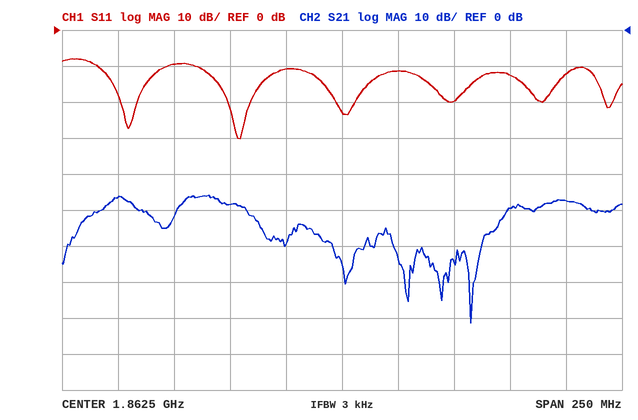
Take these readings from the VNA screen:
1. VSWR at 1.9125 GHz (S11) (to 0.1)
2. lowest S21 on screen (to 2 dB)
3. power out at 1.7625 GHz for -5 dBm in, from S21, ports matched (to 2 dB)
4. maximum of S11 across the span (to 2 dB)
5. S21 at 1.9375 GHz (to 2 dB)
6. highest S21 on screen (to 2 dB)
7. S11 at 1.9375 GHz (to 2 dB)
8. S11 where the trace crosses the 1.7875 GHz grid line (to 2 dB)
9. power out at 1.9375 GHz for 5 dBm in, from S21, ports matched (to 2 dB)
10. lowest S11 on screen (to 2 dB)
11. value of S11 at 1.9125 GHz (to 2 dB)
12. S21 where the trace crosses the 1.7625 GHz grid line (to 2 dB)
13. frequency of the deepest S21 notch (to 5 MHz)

1.2
-82 dB
-52 dBm
-8 dB
-50 dB
-46 dB
-12 dB
-10 dB
-44 dBm
-30 dB
-20 dB
-46 dB
1.920 GHz
